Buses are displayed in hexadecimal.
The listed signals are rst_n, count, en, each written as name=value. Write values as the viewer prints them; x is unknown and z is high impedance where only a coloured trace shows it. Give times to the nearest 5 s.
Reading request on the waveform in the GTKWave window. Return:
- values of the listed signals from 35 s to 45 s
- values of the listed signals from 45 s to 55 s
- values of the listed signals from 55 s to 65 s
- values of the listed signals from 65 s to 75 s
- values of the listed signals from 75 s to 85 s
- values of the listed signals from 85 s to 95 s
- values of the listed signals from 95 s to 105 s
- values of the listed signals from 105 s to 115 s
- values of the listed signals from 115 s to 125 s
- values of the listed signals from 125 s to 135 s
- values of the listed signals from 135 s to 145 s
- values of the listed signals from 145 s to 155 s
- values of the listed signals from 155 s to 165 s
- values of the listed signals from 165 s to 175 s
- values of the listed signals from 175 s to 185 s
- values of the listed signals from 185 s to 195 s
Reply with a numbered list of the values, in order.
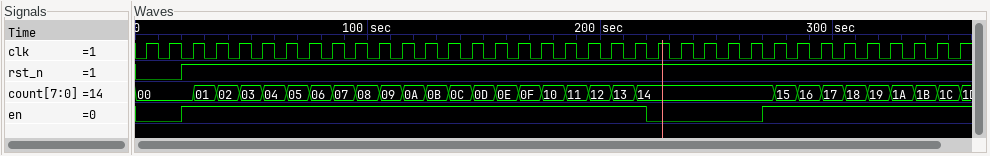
1. rst_n=1, count=02, en=1
2. rst_n=1, count=03, en=1
3. rst_n=1, count=04, en=1
4. rst_n=1, count=05, en=1
5. rst_n=1, count=06, en=1
6. rst_n=1, count=07, en=1
7. rst_n=1, count=08, en=1
8. rst_n=1, count=09, en=1
9. rst_n=1, count=0A, en=1
10. rst_n=1, count=0B, en=1
11. rst_n=1, count=0C, en=1
12. rst_n=1, count=0D, en=1
13. rst_n=1, count=0E, en=1
14. rst_n=1, count=0F, en=1
15. rst_n=1, count=10, en=1
16. rst_n=1, count=11, en=1
